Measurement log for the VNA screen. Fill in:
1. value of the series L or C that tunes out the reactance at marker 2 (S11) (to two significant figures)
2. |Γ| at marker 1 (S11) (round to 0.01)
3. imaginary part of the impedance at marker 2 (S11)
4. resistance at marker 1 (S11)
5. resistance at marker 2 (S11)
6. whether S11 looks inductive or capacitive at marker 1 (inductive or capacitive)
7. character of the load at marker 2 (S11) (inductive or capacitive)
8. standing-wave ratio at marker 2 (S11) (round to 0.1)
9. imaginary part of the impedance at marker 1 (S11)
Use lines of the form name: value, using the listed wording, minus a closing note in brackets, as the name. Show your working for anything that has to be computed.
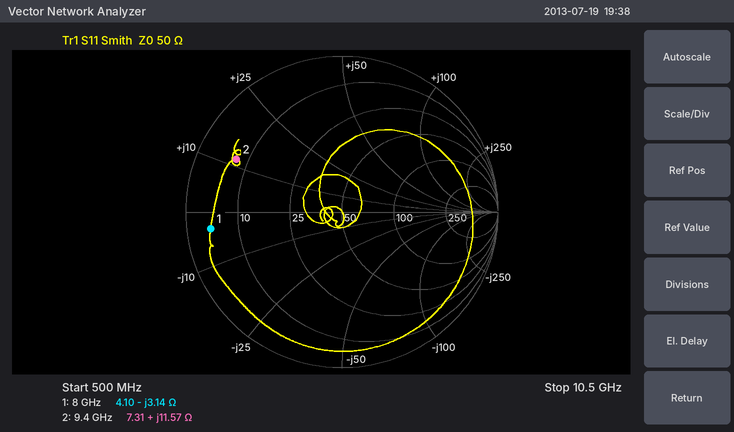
value of the series L or C that tunes out the reactance at marker 2 (S11): C = 1/(2π × 9.4 GHz × 11.57 Ω) ≈ 1.5 pF
|Γ| at marker 1 (S11): 0.85
imaginary part of the impedance at marker 2: +11.57 Ω
resistance at marker 1: 4.10 Ω
resistance at marker 2: 7.31 Ω
whether S11 looks inductive or capacitive at marker 1: capacitive
character of the load at marker 2 (S11): inductive
standing-wave ratio at marker 2 (S11): 7.2
imaginary part of the impedance at marker 1: -3.14 Ω
